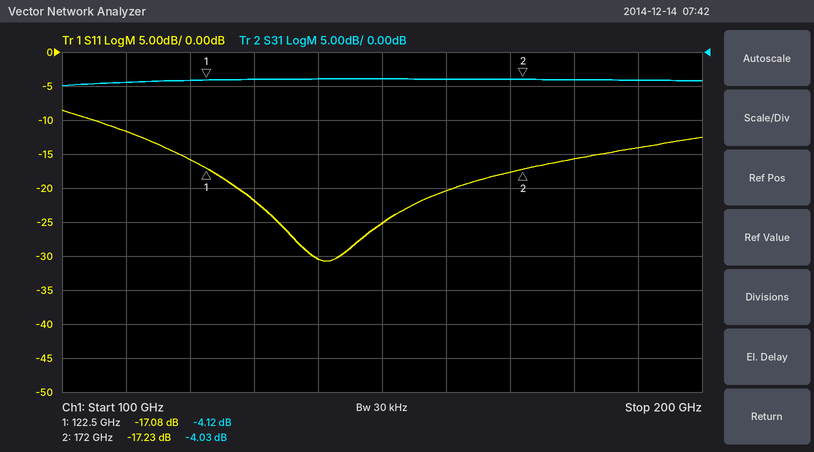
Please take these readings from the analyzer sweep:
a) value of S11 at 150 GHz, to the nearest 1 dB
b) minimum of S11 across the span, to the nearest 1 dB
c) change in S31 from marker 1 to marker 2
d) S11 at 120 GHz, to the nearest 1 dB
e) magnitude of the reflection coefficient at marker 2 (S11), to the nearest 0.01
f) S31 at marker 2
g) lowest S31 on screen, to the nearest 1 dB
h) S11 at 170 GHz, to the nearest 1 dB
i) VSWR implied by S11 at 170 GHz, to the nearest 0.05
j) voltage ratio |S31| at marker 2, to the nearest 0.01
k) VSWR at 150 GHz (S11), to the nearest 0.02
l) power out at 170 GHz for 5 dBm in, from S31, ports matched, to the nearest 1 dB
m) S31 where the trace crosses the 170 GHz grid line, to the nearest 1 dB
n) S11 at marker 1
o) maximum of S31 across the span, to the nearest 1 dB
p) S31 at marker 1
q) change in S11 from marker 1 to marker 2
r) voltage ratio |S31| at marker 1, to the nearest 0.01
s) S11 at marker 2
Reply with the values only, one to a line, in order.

-25 dB
-31 dB
0.09 dB
-16 dB
0.14
-4.03 dB
-5 dB
-18 dB
1.30
0.63
1.12
1 dBm
-4 dB
-17.08 dB
-4 dB
-4.12 dB
-0.15 dB
0.62
-17.23 dB
